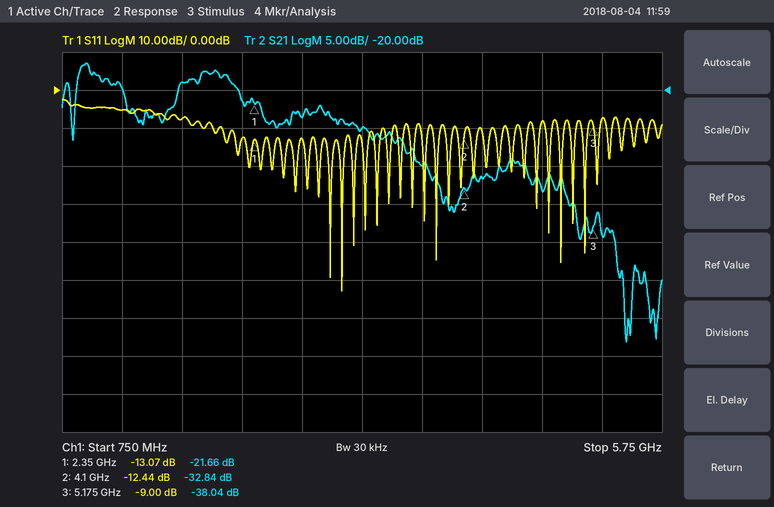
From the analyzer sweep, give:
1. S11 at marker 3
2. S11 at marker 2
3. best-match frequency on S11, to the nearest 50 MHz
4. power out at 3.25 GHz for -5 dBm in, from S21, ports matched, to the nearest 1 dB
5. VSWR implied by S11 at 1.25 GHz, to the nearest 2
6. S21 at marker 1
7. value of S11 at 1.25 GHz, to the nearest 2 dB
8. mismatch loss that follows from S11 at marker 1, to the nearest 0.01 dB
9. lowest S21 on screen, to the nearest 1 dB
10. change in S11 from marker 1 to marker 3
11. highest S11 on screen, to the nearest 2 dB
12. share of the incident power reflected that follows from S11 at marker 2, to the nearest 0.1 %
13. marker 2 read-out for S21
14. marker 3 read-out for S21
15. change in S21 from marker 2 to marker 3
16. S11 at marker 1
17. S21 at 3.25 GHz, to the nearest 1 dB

-9.00 dB
-12.44 dB
3.10 GHz
-30 dBm
4
-21.66 dB
-6 dB
0.22 dB
-53 dB
4.07 dB
-2 dB
5.7 %
-32.84 dB
-38.04 dB
-5.20 dB
-13.07 dB
-25 dB
